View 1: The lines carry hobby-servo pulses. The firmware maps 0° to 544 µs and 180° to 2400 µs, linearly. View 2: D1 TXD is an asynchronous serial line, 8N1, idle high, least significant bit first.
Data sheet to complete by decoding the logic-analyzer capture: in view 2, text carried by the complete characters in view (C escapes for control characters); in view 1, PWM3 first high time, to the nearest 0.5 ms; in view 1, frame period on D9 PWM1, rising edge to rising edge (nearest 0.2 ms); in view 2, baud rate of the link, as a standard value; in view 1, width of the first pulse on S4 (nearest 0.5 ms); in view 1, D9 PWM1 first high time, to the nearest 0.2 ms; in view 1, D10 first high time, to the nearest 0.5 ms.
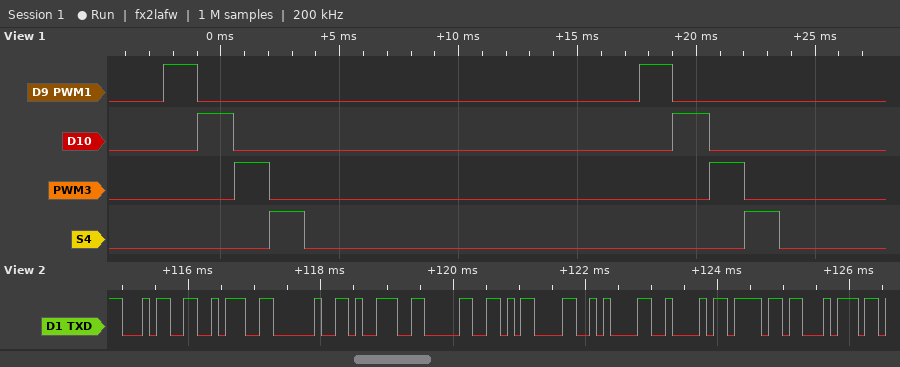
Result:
"4: 90\r\nBot"
1.5 ms
20.0 ms
9600 baud
1.5 ms
1.4 ms
1.5 ms
